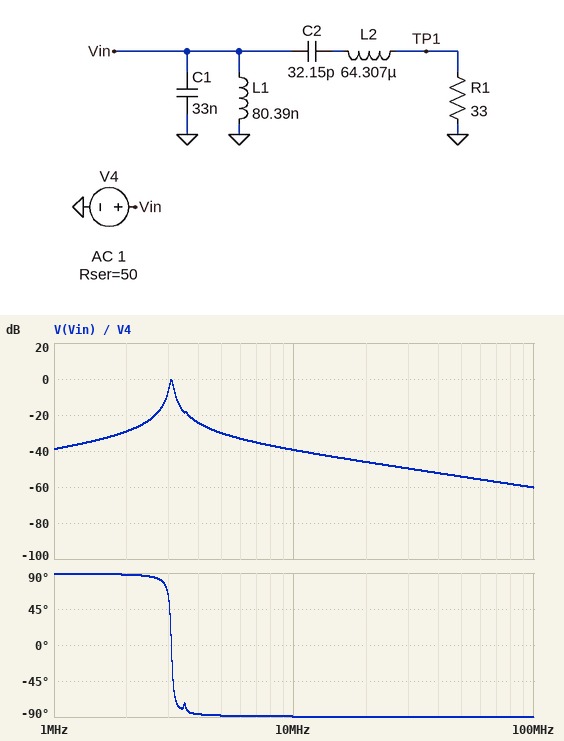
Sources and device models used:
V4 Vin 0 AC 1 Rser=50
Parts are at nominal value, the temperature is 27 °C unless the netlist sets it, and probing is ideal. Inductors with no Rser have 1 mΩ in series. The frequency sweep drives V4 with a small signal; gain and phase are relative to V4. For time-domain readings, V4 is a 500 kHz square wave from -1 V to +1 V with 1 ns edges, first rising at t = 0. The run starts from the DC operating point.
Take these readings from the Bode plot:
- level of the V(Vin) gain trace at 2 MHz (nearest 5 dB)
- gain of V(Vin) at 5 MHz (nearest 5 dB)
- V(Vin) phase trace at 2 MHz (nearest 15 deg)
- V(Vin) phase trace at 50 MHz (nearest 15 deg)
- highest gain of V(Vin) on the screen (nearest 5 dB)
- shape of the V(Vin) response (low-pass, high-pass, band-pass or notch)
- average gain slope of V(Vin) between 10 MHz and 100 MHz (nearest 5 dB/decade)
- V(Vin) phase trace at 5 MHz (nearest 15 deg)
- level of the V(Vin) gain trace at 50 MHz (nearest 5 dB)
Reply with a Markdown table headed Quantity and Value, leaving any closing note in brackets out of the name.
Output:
| Quantity | Value |
|---|---|
| level of the V(Vin) gain trace at 2 MHz | -30 dB |
| gain of V(Vin) at 5 MHz | -30 dB |
| V(Vin) phase trace at 2 MHz | 90 deg |
| V(Vin) phase trace at 50 MHz | -90 deg |
| highest gain of V(Vin) on the screen | 0 dB |
| shape of the V(Vin) response | band-pass |
| average gain slope of V(Vin) between 10 MHz and 100 MHz | -20 dB/decade |
| V(Vin) phase trace at 5 MHz | -90 deg |
| level of the V(Vin) gain trace at 50 MHz | -55 dB |
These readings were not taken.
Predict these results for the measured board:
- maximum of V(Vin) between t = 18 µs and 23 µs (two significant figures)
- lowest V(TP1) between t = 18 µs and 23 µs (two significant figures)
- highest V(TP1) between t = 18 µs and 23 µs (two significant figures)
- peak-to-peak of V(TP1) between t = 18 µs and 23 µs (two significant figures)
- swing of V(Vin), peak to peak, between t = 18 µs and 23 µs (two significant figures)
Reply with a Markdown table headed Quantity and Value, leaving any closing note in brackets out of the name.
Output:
| Quantity | Value |
|---|---|
| maximum of V(Vin) between t = 18 µs and 23 µs | 39 mV |
| lowest V(TP1) between t = 18 µs and 23 µs | -22 mV |
| highest V(TP1) between t = 18 µs and 23 µs | 22 mV |
| peak-to-peak of V(TP1) between t = 18 µs and 23 µs | 44 mV |
| swing of V(Vin), peak to peak, between t = 18 µs and 23 µs | 79 mV |
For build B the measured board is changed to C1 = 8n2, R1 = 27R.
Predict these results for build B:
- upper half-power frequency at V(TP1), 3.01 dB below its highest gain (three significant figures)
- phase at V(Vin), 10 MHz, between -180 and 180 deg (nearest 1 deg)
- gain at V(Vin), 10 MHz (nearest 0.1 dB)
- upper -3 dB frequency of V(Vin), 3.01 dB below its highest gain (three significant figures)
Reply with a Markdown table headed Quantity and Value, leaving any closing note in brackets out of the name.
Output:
| Quantity | Value |
|---|---|
| upper half-power frequency at V(TP1), 3.01 dB below its highest gain | 3.53 MHz |
| phase at V(Vin), 10 MHz, between -180 and 180 deg | -86 deg |
| gain at V(Vin), 10 MHz | -24.0 dB |
| upper -3 dB frequency of V(Vin), 3.01 dB below its highest gain | 6.40 MHz |
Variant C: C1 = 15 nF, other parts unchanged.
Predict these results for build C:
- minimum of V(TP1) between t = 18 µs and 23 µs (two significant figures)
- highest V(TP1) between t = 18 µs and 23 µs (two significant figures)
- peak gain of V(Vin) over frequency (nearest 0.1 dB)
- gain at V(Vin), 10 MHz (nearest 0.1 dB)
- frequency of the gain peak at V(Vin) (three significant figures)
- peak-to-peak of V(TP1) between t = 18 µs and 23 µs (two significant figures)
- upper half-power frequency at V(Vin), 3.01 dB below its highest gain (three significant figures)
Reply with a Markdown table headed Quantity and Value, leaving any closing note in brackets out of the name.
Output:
| Quantity | Value |
|---|---|
| minimum of V(TP1) between t = 18 µs and 23 µs | -20 mV |
| highest V(TP1) between t = 18 µs and 23 µs | 20 mV |
| peak gain of V(Vin) over frequency | -0.1 dB |
| gain at V(Vin), 10 MHz | -31.4 dB |
| frequency of the gain peak at V(Vin) | 4.59 MHz |
| peak-to-peak of V(TP1) between t = 18 µs and 23 µs | 41 mV |
| upper half-power frequency at V(Vin), 3.01 dB below its highest gain | 4.70 MHz |
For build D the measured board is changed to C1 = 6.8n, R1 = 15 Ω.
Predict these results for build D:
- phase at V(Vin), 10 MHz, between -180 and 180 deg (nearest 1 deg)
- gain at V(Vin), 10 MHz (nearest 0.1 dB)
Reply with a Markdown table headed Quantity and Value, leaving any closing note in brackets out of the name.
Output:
| Quantity | Value |
|---|---|
| phase at V(Vin), 10 MHz, between -180 and 180 deg | -85 deg |
| gain at V(Vin), 10 MHz | -21.2 dB |
